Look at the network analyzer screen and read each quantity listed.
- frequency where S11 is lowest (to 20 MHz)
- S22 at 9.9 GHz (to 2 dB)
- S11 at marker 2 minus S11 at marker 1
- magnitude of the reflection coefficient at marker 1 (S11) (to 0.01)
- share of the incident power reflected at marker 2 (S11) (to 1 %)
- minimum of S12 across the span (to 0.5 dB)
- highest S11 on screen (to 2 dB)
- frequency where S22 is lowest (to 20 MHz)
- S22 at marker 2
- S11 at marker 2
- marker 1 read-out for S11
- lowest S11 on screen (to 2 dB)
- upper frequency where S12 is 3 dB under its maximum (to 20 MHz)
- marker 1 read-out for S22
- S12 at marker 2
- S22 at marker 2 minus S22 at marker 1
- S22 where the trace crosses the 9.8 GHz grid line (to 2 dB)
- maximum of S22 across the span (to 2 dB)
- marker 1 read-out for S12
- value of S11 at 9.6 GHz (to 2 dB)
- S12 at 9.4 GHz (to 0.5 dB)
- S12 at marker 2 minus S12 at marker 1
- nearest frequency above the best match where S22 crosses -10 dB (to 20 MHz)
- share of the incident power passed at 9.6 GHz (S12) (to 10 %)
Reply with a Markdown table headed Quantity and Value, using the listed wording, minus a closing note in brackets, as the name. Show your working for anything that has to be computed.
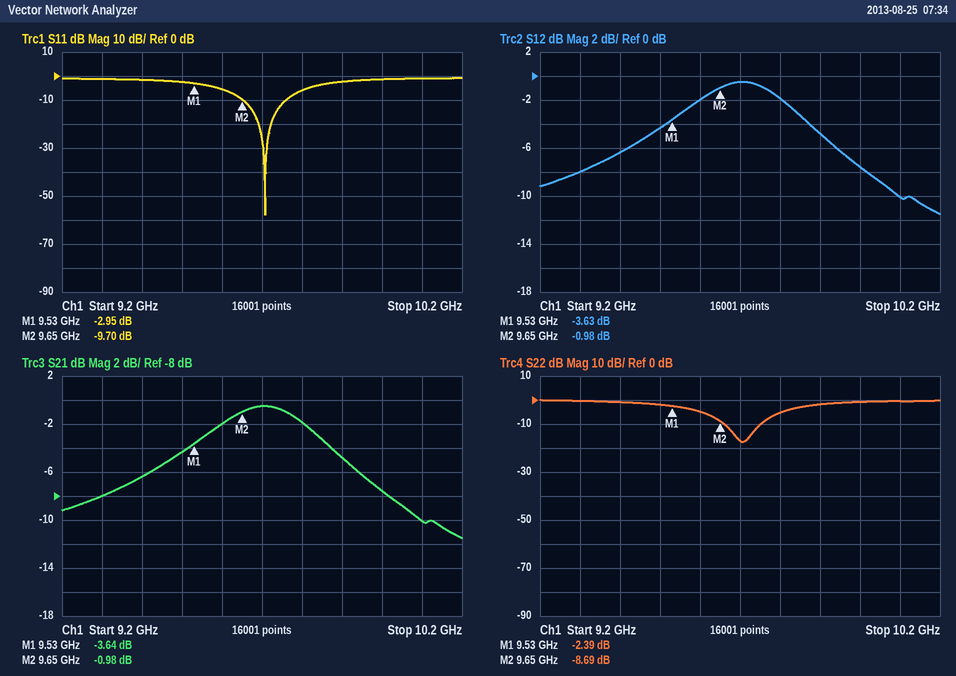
| Quantity | Value |
|---|---|
| frequency where S11 is lowest | 9.70 GHz |
| S22 at 9.9 GHz | -2 dB |
| S11 at marker 2 minus S11 at marker 1 | -9.7 − (-2.95) = -6.75 dB |
| magnitude of the reflection coefficient at marker 1 (S11) | 10^(-2.95/20) ≈ 0.71 |
| share of the incident power reflected at marker 2 (S11) | 10^(-9.7/10) ≈ 11 % |
| minimum of S12 across the span | -11.5 dB |
| highest S11 on screen | 0 dB |
| frequency where S22 is lowest | 9.70 GHz |
| S22 at marker 2 | -8.69 dB |
| S11 at marker 2 | -9.70 dB |
| marker 1 read-out for S11 | -2.95 dB |
| lowest S11 on screen | -58 dB |
| upper frequency where S12 is 3 dB under its maximum | 9.86 GHz |
| marker 1 read-out for S22 | -2.39 dB |
| S12 at marker 2 | -0.98 dB |
| S22 at marker 2 minus S22 at marker 1 | -8.69 − (-2.39) = -6.30 dB |
| S22 where the trace crosses the 9.8 GHz grid line | -6 dB |
| maximum of S22 across the span | 0 dB |
| marker 1 read-out for S12 | -3.63 dB |
| value of S11 at 9.6 GHz | -6 dB |
| S12 at 9.4 GHz | -6.5 dB |
| S12 at marker 2 minus S12 at marker 1 | -0.98 − (-3.63) = 2.65 dB |
| nearest frequency above the best match where S22 crosses -10 dB | 9.76 GHz |
| share of the incident power passed at 9.6 GHz (S12) | 10^(-2/10) ≈ 63.1 %, so 60 % to the nearest 10 % |
